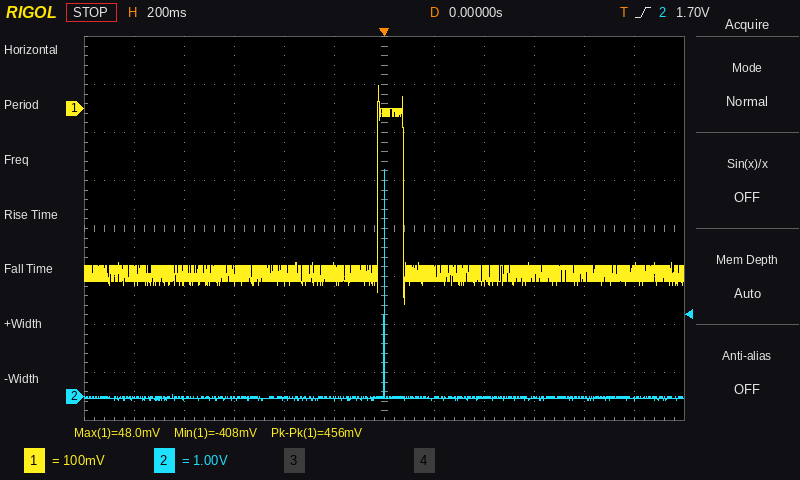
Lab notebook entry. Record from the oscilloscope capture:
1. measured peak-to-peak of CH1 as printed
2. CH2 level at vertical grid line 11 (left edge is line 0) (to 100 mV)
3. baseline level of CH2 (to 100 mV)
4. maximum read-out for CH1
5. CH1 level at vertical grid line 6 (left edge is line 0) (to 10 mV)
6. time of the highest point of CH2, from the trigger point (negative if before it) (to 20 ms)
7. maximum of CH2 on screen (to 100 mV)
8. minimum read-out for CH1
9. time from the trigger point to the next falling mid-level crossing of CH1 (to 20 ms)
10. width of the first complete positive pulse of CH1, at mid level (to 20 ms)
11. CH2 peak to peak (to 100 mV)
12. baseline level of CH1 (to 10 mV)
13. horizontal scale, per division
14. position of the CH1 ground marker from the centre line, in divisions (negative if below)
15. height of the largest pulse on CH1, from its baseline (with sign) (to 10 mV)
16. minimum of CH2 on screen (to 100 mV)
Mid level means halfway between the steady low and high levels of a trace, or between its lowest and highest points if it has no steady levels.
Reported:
456 mV
0.0 V
0.0 V
48.0 mV
-10 mV
0 ms
4.7 V
-408 mV
80 ms
100 ms
4.8 V
-340 mV
200 ms
+2.5 div
+390 mV
-100 mV
